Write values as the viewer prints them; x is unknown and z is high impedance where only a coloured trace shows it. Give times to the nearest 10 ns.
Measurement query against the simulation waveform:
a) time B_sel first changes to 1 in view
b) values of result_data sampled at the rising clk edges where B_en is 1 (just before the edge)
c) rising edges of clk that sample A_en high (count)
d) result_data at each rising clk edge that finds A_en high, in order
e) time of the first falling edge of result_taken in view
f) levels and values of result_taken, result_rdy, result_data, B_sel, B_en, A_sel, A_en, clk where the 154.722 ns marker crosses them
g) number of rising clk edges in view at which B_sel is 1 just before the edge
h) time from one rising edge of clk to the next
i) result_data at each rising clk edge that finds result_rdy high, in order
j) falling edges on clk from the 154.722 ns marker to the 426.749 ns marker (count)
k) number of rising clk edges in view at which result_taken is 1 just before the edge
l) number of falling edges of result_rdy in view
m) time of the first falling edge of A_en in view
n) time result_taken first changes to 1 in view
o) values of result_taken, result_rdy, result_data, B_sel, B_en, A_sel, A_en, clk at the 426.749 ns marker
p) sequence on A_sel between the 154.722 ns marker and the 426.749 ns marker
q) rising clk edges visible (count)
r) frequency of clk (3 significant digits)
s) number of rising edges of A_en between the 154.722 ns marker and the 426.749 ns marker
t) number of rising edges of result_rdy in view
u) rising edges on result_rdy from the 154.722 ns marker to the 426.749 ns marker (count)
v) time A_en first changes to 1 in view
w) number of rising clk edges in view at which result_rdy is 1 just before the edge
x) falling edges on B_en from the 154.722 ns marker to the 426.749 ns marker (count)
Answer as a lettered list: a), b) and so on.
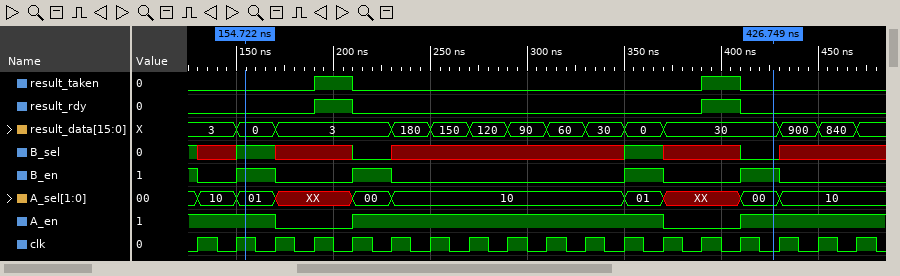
a) 150 ns
b) 3, 0, 3, 0, 30
c) 14
d) 3, 3, 0, 3, 180, 150, 120, 90, 60, 30, 0, 30, 900, 840
e) 210 ns
f) result_taken=0, result_rdy=0, result_data=0, B_sel=1, B_en=1, A_sel=01, A_en=1, clk=1
g) 3
h) 20 ns
i) 3, 30
j) 14
k) 2
l) 2
m) 170 ns
n) 190 ns
o) result_taken=0, result_rdy=0, result_data=30, B_sel=0, B_en=1, A_sel=00, A_en=1, clk=0
p) 01, XX, 00, 10, 01, XX, 00
q) 18
r) 50.0 MHz
s) 2
t) 2
u) 2
v) 210 ns
w) 2
x) 3
